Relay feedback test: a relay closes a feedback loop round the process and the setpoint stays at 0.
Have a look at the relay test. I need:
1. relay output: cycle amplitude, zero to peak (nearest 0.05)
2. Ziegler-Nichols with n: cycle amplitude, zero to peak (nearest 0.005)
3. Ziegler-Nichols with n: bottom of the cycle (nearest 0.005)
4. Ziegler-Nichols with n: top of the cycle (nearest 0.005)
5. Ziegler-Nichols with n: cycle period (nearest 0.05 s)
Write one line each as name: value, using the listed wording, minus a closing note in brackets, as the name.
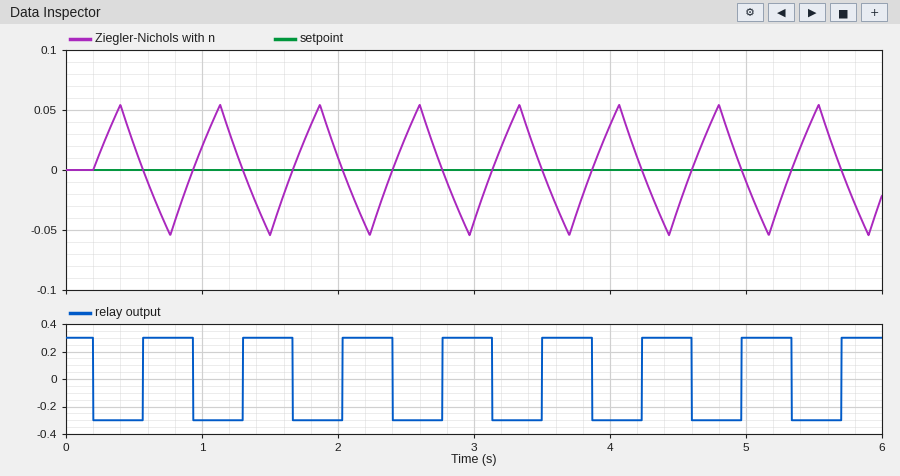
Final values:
relay output: cycle amplitude, zero to peak: 0.30
Ziegler-Nichols with n: cycle amplitude, zero to peak: 0.055
Ziegler-Nichols with n: bottom of the cycle: -0.055
Ziegler-Nichols with n: top of the cycle: 0.055
Ziegler-Nichols with n: cycle period: 0.75 s
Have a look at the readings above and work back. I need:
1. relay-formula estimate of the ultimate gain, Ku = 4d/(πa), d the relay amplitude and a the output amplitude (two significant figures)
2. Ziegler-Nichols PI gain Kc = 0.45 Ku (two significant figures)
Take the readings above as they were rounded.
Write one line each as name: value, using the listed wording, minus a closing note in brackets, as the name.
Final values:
relay-formula estimate of the ultimate gain, Ku = 4d/(πa), d the relay amplitude and a the output amplitude: 6.9
Ziegler-Nichols PI gain Kc = 0.45 Ku: 3.1
